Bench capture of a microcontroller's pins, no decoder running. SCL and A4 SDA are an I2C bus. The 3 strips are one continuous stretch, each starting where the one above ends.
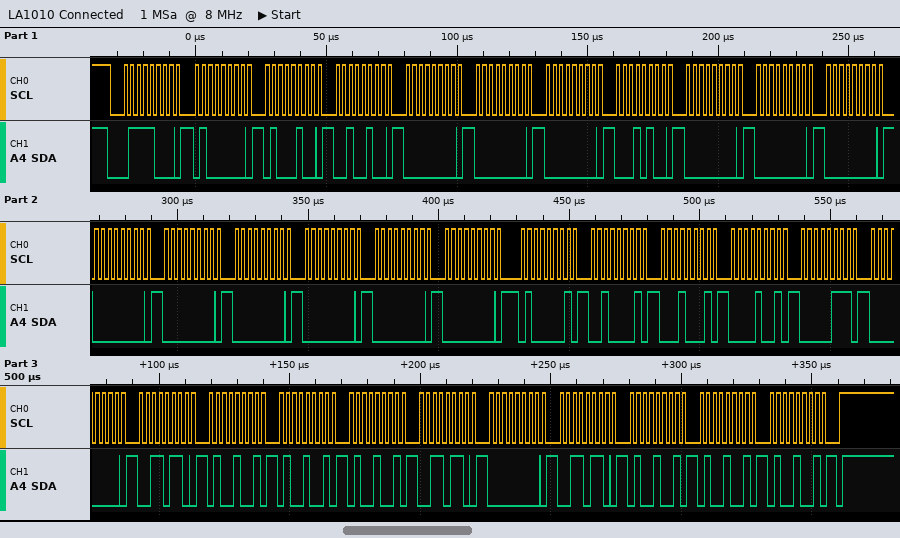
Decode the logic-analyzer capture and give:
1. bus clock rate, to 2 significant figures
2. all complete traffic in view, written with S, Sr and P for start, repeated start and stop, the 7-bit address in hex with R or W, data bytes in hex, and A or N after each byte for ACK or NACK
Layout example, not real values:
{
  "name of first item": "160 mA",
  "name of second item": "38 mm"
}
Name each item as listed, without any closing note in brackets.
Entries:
{
  "bus clock rate, to 2 significant figures": "400 kHz",
  "all complete traffic in view, written with S, Sr and P for start, repeated start and stop, the 7-bit address in hex with R or W, data bytes in hex, and A or N after each byte for ACK or NACK": "S 3CW A 40 A 44 A 24 A 00 A 00 A 00 A 14 A 00 A 00 A 00 A 00 A 00 A 00 A 00 A 00 A 00 A 41 A 21 A 11 A 09 A 07 A 00 A 36 A 49 A 49 A 49 A 36 A 00 A 36 A 49 A 49 A 49 A P"
}
